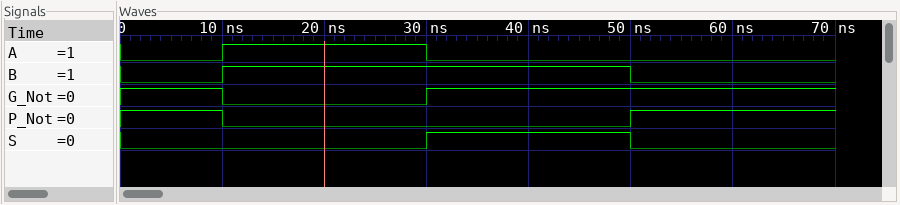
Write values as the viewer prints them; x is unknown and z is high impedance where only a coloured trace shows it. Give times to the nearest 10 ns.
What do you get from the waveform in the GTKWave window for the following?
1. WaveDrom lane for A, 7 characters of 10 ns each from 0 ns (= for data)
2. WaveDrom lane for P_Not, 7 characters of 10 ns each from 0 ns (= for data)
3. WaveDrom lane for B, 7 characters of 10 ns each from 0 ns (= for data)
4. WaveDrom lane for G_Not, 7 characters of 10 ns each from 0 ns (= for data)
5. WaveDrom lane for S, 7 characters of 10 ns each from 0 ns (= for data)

{name: 'A', wave: '01.0...'}
{name: 'P_Not', wave: '10...1.'}
{name: 'B', wave: '01...0.'}
{name: 'G_Not', wave: '10.1...'}
{name: 'S', wave: '0..1.0.'}
